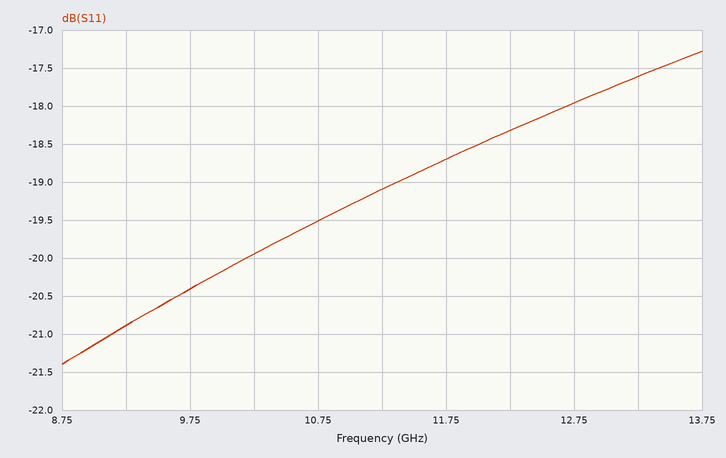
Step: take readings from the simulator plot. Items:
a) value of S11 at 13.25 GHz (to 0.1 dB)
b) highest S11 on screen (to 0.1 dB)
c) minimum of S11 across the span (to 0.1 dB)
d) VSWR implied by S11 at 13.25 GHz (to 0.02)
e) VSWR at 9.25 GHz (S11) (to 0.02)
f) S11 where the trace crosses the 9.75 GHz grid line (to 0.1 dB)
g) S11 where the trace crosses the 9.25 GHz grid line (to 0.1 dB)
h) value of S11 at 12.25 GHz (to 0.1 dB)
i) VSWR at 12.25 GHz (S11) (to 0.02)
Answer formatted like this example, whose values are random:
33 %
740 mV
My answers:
-17.6 dB
-17.3 dB
-21.4 dB
1.30
1.20
-20.4 dB
-20.9 dB
-18.3 dB
1.28
